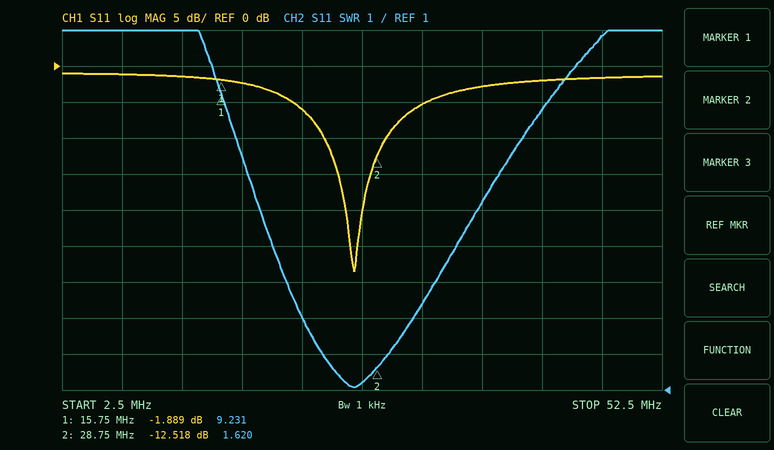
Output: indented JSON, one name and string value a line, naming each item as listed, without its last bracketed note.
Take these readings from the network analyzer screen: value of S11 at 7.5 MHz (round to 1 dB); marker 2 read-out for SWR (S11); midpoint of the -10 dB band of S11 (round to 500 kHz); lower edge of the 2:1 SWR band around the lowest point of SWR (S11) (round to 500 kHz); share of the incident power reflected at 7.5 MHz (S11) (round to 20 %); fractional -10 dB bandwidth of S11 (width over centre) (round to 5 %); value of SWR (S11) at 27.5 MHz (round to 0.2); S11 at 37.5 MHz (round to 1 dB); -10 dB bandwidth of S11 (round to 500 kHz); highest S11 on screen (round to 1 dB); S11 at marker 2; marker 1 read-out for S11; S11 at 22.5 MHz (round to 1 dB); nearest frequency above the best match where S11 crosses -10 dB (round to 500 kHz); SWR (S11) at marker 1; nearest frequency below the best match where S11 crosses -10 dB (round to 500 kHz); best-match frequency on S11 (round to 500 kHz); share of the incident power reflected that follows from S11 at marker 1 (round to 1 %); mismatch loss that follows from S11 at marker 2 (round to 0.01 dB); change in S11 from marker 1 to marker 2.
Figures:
{
  "value of S11 at 7.5 MHz": "-1 dB",
  "marker 2 read-out for SWR": "1.620",
  "midpoint of the -10 dB band of S11": "27.0 MHz",
  "lower edge of the 2:1 SWR band around the lowest point of SWR (S11)": "24.0 MHz",
  "share of the incident power reflected at 7.5 MHz (S11)": "80 %",
  "fractional -10 dB bandwidth of S11 (width over centre)": "20 %",
  "value of SWR (S11) at 27.5 MHz": "1.2",
  "S11 at 37.5 MHz": "-3 dB",
  "-10 dB bandwidth of S11": "5.0 MHz",
  "highest S11 on screen": "-1 dB",
  "S11 at marker 2": "-12.518 dB",
  "marker 1 read-out for S11": "-1.889 dB",
  "S11 at 22.5 MHz": "-6 dB",
  "nearest frequency above the best match where S11 crosses -10 dB": "29.5 MHz",
  "SWR (S11) at marker 1": "9.231",
  "nearest frequency below the best match where S11 crosses -10 dB": "24.5 MHz",
  "best-match frequency on S11": "27.0 MHz",
  "share of the incident power reflected that follows from S11 at marker 1": "65 %",
  "mismatch loss that follows from S11 at marker 2": "0.25 dB",
  "change in S11 from marker 1 to marker 2": "-10.629 dB"
}
